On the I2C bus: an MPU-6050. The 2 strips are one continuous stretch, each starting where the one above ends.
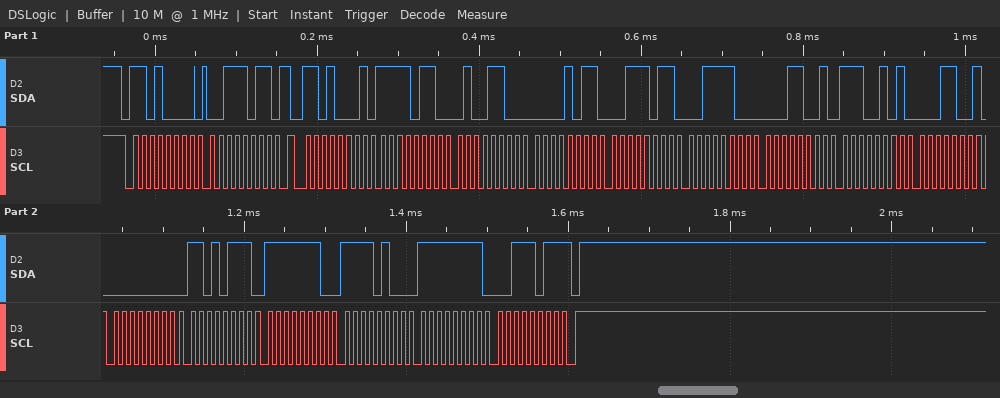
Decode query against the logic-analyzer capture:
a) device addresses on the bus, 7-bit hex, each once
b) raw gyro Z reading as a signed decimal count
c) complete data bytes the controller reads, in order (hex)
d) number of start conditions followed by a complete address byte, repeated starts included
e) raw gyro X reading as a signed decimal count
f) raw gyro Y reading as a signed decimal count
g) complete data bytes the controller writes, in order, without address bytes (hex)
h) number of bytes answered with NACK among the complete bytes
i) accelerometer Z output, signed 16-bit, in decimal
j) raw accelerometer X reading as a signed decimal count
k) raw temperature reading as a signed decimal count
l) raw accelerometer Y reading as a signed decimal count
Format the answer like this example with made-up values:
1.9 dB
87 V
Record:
0x68
-197
F6 4C 0B 3B 3C 19 E5 19 00 D7 FE F4 FF 3B
2
215
-268
3B
1
15385
-2484
-6887
2875
